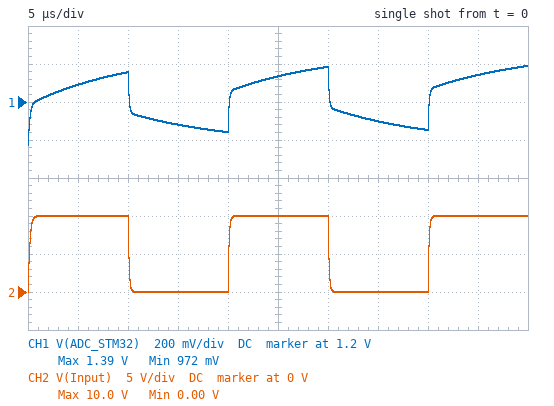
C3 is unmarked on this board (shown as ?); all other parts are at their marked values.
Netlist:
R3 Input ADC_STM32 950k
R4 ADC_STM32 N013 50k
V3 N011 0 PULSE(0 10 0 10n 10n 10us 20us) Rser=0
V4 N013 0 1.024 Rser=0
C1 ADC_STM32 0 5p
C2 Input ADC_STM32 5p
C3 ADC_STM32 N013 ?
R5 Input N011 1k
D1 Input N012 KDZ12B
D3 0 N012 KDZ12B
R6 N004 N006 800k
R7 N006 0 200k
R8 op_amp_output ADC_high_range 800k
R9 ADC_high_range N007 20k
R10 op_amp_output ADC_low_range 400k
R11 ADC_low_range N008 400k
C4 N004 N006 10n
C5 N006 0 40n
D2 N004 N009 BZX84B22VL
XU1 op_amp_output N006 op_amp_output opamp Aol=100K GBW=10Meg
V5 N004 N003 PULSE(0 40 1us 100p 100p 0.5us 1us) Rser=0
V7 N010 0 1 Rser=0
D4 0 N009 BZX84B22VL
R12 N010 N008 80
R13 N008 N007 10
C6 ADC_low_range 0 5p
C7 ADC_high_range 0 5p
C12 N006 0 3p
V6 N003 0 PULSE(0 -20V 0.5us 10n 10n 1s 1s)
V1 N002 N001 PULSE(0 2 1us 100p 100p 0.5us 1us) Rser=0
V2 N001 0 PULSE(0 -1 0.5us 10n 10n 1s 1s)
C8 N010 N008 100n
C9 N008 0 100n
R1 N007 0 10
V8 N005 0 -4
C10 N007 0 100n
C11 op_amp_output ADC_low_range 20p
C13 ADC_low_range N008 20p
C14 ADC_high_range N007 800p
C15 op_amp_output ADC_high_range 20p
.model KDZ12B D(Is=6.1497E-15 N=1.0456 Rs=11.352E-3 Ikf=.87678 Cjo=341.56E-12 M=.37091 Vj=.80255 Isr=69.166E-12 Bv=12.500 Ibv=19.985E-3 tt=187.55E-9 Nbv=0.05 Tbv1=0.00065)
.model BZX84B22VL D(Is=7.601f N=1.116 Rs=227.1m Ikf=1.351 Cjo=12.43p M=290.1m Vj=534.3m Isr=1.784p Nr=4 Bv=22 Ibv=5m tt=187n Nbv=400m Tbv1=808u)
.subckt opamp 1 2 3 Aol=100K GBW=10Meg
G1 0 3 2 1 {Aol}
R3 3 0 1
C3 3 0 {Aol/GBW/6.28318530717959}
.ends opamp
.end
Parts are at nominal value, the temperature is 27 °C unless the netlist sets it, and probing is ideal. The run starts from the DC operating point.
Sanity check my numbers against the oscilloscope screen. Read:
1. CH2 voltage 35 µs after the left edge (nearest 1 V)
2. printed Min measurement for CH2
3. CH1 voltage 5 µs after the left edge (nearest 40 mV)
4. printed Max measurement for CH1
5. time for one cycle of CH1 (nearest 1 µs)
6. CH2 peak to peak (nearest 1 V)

0 V
0.00 V
1.28 V
1.39 V
20 µs
10 V
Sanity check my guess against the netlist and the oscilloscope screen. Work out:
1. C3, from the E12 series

220 pF
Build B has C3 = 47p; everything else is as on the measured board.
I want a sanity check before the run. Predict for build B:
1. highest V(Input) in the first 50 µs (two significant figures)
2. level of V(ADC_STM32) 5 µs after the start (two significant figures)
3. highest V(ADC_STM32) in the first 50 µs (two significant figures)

10 V
1.5 V
1.8 V
